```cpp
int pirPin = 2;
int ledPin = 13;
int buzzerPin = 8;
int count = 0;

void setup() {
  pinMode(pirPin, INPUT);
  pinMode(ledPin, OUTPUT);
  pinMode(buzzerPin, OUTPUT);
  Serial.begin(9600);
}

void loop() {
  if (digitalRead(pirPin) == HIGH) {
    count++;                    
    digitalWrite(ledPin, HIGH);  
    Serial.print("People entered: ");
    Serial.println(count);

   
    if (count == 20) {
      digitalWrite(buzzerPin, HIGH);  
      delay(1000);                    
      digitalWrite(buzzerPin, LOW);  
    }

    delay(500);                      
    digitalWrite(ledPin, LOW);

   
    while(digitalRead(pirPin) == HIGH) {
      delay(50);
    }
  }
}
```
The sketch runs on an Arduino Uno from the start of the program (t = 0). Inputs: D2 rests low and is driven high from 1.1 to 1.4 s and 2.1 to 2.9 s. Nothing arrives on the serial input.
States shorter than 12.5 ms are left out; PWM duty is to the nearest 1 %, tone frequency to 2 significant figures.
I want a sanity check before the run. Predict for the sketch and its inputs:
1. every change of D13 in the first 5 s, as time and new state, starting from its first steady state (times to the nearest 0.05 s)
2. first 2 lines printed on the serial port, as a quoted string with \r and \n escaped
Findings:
0 s low; 1.1 s high; 1.6 s low; 2.1 s high; 2.6 s low
"People entered: 1\r\nPeople entered: 2\r\n"
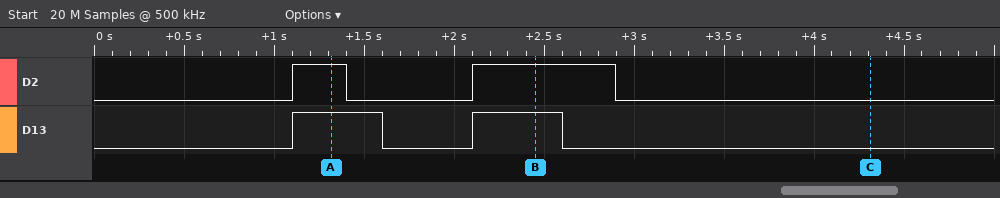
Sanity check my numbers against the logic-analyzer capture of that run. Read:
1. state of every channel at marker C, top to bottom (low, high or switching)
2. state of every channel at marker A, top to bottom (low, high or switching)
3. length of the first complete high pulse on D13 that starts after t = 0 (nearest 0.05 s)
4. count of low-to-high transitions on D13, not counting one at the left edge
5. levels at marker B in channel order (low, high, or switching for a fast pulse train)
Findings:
D2 low, D13 low
D2 high, D13 high
0.50 s
2
D2 high, D13 high
